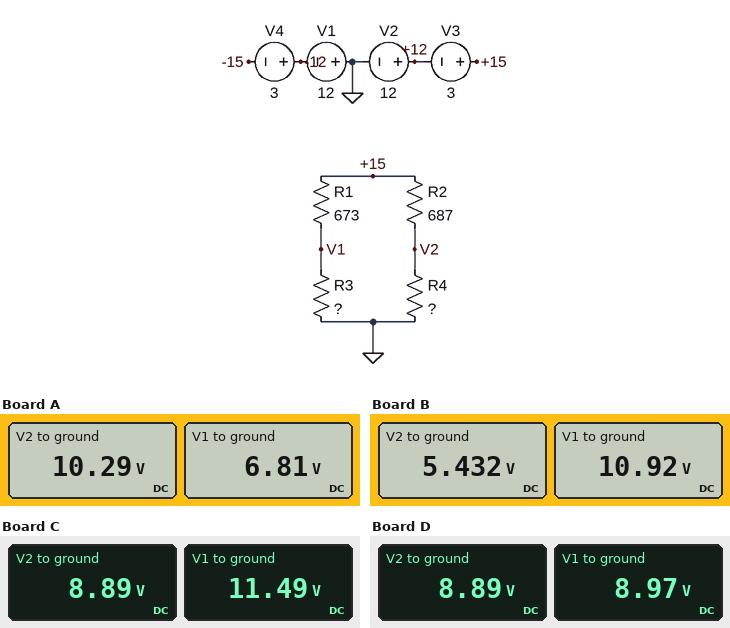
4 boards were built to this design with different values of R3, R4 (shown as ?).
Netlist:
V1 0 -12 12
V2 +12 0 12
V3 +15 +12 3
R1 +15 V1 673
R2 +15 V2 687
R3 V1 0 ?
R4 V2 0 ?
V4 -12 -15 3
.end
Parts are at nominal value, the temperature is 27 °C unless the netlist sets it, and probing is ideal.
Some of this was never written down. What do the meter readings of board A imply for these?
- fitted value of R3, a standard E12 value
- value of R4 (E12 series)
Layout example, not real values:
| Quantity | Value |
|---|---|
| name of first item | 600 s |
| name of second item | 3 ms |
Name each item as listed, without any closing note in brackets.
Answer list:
| Quantity | Value |
|---|---|
| fitted value of R3, a standard E12 value | 560 Ω |
| value of R4 | 1.5 kΩ |
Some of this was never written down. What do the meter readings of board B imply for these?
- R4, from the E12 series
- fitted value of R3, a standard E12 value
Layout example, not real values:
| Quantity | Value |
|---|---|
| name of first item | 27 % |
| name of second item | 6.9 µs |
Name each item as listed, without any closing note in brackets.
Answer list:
| Quantity | Value |
|---|---|
| R4, from the E12 series | 390 Ω |
| fitted value of R3, a standard E12 value | 1.8 kΩ |
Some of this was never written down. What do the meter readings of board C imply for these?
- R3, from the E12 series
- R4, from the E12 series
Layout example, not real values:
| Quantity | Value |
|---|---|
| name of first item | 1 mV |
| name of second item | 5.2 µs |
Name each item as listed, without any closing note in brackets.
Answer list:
| Quantity | Value |
|---|---|
| R3, from the E12 series | 2.2 kΩ |
| R4, from the E12 series | 1 kΩ |
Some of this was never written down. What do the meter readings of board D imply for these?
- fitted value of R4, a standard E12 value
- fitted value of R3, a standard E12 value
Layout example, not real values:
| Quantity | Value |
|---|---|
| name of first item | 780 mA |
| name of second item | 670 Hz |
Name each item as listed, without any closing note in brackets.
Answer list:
| Quantity | Value |
|---|---|
| fitted value of R4, a standard E12 value | 1 kΩ |
| fitted value of R3, a standard E12 value | 1 kΩ |
